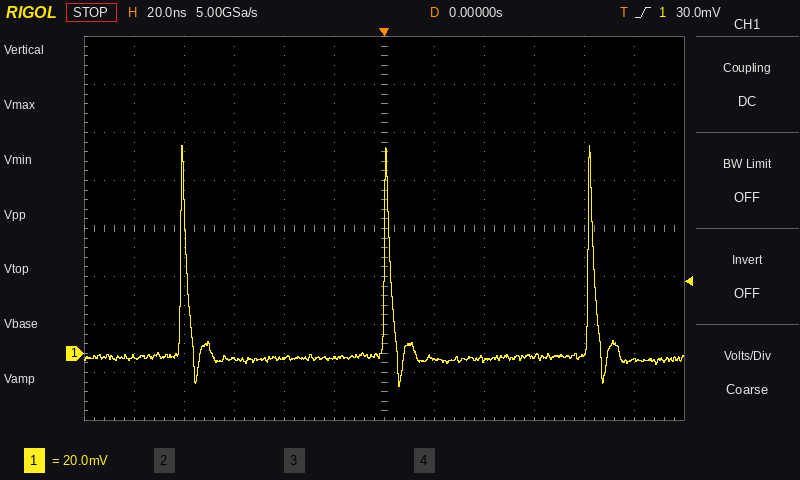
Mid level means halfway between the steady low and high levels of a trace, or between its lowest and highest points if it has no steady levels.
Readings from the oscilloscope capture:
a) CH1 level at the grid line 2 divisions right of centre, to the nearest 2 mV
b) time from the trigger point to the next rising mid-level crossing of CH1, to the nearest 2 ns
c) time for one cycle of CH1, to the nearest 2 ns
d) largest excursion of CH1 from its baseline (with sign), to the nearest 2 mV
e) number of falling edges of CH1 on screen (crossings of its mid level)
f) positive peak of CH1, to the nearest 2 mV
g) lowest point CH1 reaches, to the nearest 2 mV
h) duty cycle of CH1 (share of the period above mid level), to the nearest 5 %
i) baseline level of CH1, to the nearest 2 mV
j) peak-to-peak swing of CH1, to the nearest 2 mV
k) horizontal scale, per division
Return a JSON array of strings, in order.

["-2 mV", "82 ns", "82 ns", "+88 mV", "3", "86 mV", "-14 mV", "5 %", "-2 mV", "100 mV", "20 ns"]
